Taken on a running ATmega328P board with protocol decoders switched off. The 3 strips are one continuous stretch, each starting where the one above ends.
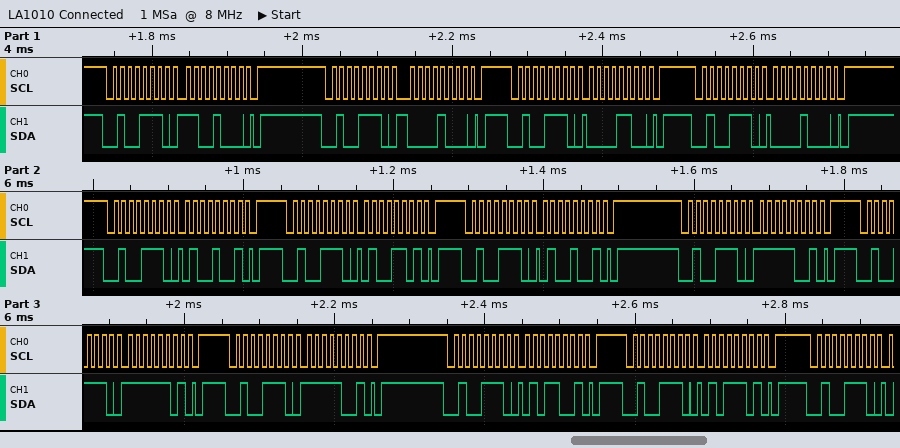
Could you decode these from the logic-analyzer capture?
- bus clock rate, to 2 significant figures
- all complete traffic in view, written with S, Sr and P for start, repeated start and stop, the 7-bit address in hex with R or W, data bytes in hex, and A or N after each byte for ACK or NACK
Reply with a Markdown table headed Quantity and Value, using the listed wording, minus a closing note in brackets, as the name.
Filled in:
| Quantity | Value |
|---|---|
| bus clock rate, to 2 significant figures | 100 kHz |
| all complete traffic in view, written with S, Sr and P for start, repeated start and stop, the 7-bit address in hex with R or W, data bytes in hex, and A or N after each byte for ACK or NACK | S 27W A C8 A P S 27W A 08 A P S 27W A 0C A P S 27W A 08 A P S 27W A 49 A P S 27W A 4D A P S 27W A 49 A P S 27W A F9 A P S 27W A FD A P S 27W A F9 A P S 27W A 59 A P S 27W A 5D A P S 27W A |
